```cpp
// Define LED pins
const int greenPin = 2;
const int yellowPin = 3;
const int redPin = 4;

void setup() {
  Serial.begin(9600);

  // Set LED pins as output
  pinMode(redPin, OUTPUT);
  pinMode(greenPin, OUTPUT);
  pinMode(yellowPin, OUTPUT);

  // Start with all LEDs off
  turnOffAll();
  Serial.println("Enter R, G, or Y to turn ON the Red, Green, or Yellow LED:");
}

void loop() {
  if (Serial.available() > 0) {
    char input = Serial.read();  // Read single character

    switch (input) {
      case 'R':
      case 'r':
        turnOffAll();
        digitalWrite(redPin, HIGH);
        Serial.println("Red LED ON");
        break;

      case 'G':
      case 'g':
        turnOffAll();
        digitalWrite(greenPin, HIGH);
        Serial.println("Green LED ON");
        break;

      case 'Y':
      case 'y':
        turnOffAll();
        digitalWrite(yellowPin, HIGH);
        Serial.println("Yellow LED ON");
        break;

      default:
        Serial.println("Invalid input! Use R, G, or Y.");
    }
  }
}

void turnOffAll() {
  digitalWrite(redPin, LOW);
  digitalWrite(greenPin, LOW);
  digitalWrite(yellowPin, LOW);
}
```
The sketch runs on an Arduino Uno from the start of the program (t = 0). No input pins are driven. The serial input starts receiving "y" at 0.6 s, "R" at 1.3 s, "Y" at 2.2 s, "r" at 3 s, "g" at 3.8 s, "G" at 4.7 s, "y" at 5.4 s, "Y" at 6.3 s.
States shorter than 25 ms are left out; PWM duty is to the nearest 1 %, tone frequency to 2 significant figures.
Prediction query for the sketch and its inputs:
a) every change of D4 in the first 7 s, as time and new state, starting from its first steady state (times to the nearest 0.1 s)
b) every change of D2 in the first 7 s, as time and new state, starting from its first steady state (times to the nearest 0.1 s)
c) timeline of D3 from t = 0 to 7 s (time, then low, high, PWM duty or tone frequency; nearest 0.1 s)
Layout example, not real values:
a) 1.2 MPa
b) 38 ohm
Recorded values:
a) 0 s low; 1.3 s high; 2.2 s low; 3 s high; 3.8 s low
b) 0 s low; 3.8 s high; 5.4 s low
c) 0 s low; 0.6 s high; 1.3 s low; 2.2 s high; 3 s low; 5.4 s high
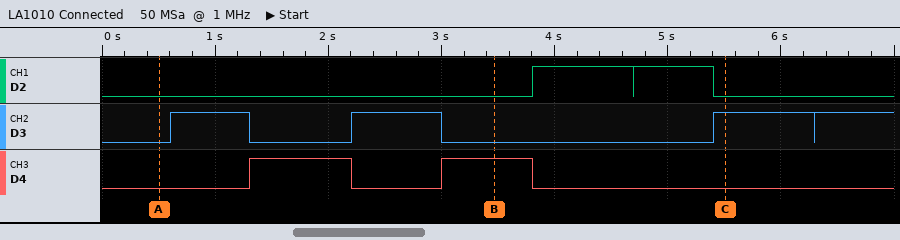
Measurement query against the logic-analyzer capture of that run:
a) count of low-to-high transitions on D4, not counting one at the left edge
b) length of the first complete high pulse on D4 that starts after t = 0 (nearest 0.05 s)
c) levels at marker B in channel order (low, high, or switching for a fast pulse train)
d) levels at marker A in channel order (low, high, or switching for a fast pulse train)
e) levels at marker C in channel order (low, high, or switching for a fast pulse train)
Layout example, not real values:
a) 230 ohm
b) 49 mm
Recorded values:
a) 2
b) 0.90 s
c) D2 low, D3 low, D4 high
d) D2 low, D3 low, D4 low
e) D2 low, D3 high, D4 low
